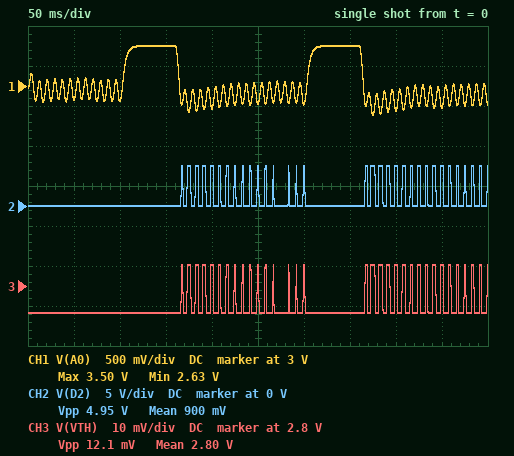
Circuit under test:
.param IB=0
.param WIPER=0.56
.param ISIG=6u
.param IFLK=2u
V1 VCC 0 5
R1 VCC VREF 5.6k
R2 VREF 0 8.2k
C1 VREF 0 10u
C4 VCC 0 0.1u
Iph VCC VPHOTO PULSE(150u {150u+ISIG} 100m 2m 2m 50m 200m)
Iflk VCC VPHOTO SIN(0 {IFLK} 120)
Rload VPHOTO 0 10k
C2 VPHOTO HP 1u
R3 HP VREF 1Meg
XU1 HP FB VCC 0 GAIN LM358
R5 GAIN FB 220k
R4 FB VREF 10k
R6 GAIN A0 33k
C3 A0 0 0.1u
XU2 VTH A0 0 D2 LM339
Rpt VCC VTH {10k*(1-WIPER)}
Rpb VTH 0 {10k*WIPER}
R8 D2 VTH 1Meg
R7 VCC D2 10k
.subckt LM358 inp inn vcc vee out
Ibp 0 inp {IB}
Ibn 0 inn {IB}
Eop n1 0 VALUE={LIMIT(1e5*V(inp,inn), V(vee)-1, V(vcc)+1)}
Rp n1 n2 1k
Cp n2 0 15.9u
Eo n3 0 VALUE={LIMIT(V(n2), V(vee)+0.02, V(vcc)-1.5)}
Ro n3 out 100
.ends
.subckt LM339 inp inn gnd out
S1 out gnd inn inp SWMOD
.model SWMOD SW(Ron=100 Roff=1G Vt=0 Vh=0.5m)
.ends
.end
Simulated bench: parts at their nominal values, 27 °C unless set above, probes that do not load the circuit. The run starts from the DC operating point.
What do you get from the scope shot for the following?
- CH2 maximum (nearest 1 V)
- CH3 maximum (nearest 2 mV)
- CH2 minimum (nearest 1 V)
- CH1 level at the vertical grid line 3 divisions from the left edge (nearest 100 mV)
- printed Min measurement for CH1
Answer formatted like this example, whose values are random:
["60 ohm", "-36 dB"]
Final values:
["5 V", "2.806 V", "0 V", "3.5 V", "2.63 V"]
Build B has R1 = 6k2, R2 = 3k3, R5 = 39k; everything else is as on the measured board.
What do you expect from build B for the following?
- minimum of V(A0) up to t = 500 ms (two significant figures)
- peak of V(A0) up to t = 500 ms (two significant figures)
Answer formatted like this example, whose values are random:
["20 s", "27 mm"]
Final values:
["1.7 V", "2.0 V"]
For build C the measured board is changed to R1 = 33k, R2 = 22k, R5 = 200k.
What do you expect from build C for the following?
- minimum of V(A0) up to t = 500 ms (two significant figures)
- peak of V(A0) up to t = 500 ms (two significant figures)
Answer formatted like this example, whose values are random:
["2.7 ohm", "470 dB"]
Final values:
["1.6 V", "3.2 V"]
